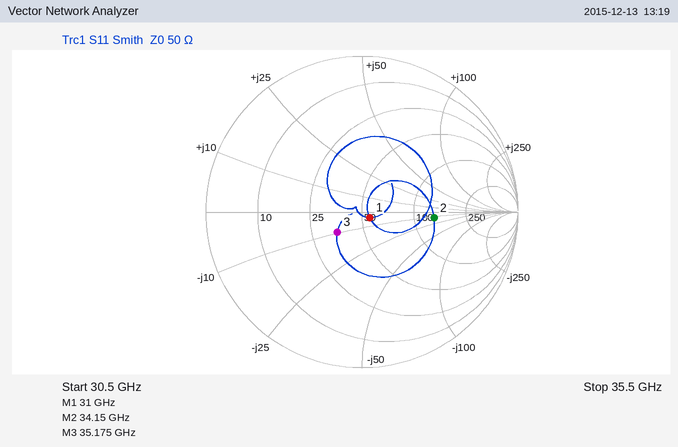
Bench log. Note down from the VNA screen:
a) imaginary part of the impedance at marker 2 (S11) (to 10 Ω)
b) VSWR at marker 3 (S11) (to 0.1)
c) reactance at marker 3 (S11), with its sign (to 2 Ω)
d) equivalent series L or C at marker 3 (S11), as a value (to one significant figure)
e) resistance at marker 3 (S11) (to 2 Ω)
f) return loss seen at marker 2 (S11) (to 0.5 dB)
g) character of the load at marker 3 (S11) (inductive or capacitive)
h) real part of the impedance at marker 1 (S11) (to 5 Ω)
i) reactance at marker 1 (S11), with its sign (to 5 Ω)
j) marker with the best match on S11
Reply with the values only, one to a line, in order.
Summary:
-10 Ω
1.5
-10 Ω
500 fF
36 Ω
6.5 dB
capacitive
55 Ω
-5 Ω
marker 1
